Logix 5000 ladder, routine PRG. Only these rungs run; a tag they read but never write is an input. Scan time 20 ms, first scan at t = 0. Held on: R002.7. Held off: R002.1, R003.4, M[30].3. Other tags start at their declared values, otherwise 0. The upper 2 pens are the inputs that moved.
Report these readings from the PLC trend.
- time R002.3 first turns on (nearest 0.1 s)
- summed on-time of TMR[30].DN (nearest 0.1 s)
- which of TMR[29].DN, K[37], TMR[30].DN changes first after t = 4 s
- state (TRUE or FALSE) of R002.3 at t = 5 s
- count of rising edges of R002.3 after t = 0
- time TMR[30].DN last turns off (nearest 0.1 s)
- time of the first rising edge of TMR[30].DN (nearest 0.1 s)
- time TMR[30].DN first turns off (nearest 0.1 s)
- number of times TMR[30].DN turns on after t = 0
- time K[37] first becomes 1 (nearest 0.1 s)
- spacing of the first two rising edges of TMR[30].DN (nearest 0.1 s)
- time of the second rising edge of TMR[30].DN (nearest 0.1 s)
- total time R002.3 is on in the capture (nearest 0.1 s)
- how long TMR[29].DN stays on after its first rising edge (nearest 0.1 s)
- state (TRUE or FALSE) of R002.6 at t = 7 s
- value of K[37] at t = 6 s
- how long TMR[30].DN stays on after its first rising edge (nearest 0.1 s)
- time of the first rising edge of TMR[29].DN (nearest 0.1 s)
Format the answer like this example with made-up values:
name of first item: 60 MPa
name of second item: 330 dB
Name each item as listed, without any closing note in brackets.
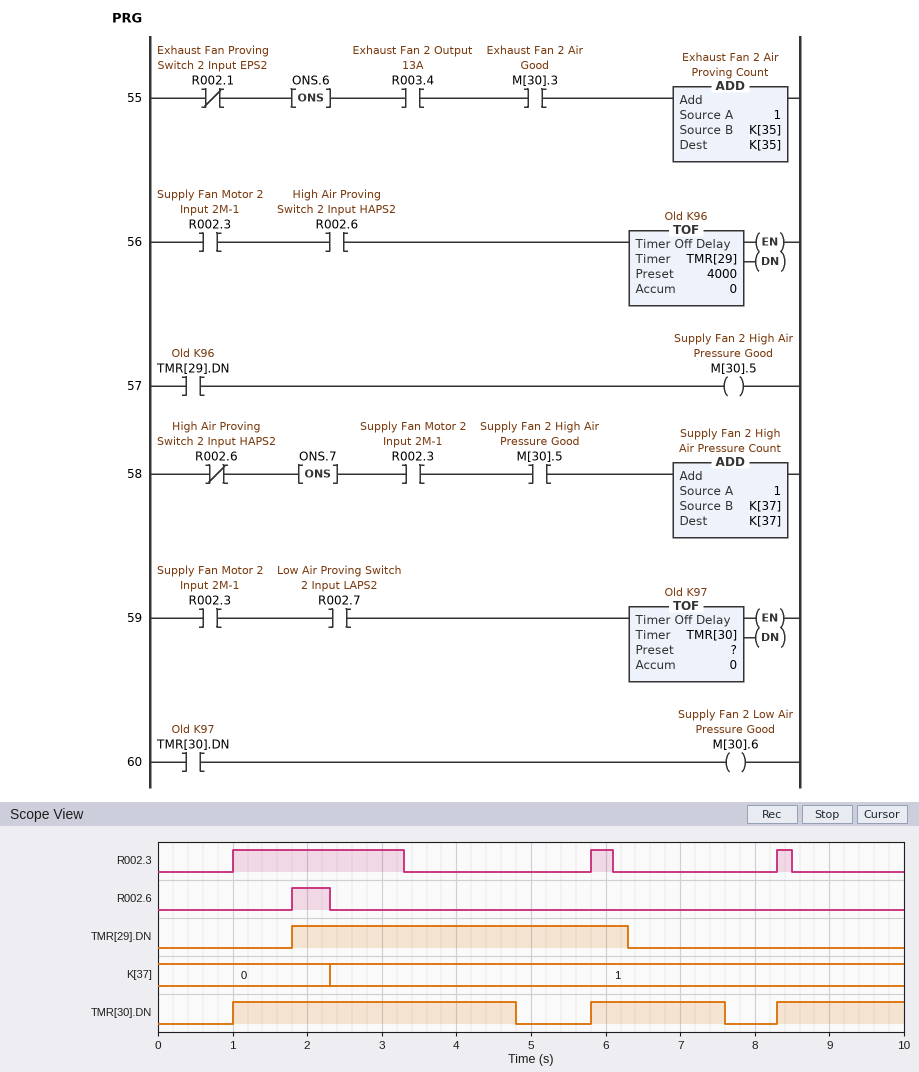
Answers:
time R002.3 first turns on: 1.0 s
summed on-time of TMR[30].DN: 7.3 s
which of TMR[29].DN, K[37], TMR[30].DN changes first after t = 4 s: TMR[30].DN
state (TRUE or FALSE) of R002.3 at t = 5 s: FALSE
count of rising edges of R002.3 after t = 0: 3
time TMR[30].DN last turns off: 7.6 s
time of the first rising edge of TMR[30].DN: 1.0 s
time TMR[30].DN first turns off: 4.8 s
number of times TMR[30].DN turns on after t = 0: 3
time K[37] first becomes 1: 2.3 s
spacing of the first two rising edges of TMR[30].DN: 4.8 s
time of the second rising edge of TMR[30].DN: 5.8 s
total time R002.3 is on in the capture: 2.8 s
how long TMR[29].DN stays on after its first rising edge: 4.5 s
state (TRUE or FALSE) of R002.6 at t = 7 s: FALSE
value of K[37] at t = 6 s: 1
how long TMR[30].DN stays on after its first rising edge: 3.8 s
time of the first rising edge of TMR[29].DN: 1.8 s
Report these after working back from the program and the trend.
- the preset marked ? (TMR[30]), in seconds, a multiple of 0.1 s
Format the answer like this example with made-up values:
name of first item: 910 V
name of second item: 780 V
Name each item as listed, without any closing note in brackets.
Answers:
the preset marked ? (TMR[30]), in seconds, a multiple of 0.1 s: 1.5 s
